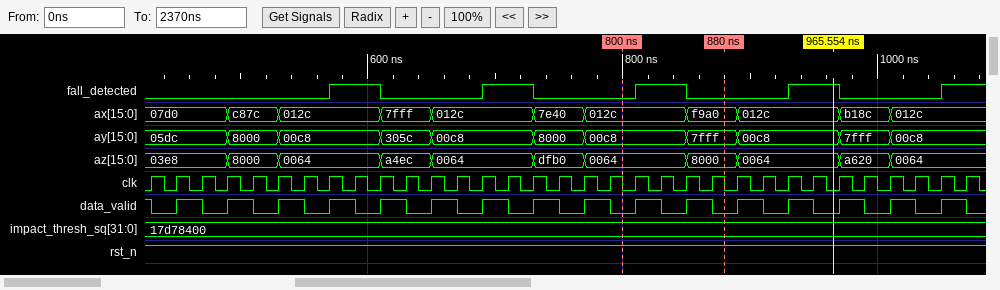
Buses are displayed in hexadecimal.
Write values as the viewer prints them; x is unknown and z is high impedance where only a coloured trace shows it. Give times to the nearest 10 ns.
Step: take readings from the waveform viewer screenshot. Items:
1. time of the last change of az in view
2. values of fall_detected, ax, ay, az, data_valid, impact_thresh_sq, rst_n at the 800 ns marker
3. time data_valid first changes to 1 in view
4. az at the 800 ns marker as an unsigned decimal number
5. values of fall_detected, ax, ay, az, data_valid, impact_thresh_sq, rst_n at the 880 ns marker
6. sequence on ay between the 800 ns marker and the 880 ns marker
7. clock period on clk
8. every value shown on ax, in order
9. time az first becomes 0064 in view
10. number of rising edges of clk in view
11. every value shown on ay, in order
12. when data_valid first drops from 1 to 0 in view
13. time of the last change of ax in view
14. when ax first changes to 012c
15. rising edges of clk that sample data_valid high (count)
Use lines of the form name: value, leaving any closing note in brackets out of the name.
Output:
time of the last change of az in view: 1010 ns
values of fall_detected, ax, ay, az, data_valid, impact_thresh_sq, rst_n at the 800 ns marker: fall_detected=0, ax=012c, ay=00c8, az=0064, data_valid=0, impact_thresh_sq=17d78400, rst_n=1
time data_valid first changes to 1 in view: 450 ns
az at the 800 ns marker as an unsigned decimal number: 100
values of fall_detected, ax, ay, az, data_valid, impact_thresh_sq, rst_n at the 880 ns marker: fall_detected=0, ax=f9a0, ay=7fff, az=8000, data_valid=0, impact_thresh_sq=17d78400, rst_n=1
sequence on ay between the 800 ns marker and the 880 ns marker: 00c8, 7fff
clock period on clk: 20 ns
every value shown on ax, in order: 07d0, c87c, 012c, 7fff, 012c, 7e40, 012c, f9a0, 012c, b18c, 012c
time az first becomes 0064 in view: 530 ns
number of rising edges of clk in view: 33
every value shown on ay, in order: 05dc, 8000, 00c8, 305c, 00c8, 8000, 00c8, 7fff, 00c8, 7fff, 00c8
when data_valid first drops from 1 to 0 in view: 430 ns
time of the last change of ax in view: 1010 ns
when ax first changes to 012c: 530 ns
rising edges of clk that sample data_valid high: 17
